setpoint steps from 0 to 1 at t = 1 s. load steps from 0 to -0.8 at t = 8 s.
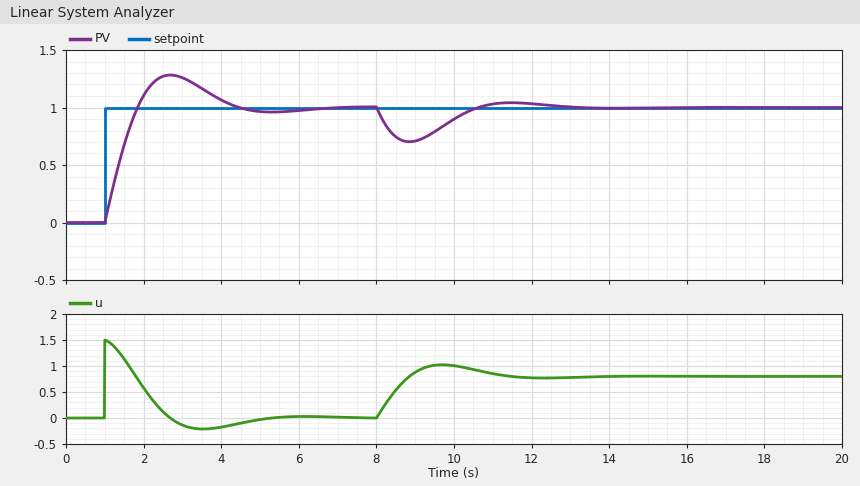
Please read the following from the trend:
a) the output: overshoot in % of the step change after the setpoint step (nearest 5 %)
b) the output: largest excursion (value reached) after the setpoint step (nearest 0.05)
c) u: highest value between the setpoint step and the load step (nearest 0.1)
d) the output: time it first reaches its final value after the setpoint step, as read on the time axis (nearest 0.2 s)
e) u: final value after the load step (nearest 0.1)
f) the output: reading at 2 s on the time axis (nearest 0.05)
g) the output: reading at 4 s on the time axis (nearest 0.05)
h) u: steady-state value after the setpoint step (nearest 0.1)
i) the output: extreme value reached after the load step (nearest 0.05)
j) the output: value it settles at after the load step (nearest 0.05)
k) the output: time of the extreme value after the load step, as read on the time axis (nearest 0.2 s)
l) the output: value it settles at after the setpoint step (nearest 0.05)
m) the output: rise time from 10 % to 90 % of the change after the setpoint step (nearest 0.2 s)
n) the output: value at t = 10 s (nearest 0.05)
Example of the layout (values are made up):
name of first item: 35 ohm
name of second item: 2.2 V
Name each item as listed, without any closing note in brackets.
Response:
the output: overshoot in % of the step change after the setpoint step: 30 %
the output: largest excursion (value reached) after the setpoint step: 1.30
u: highest value between the setpoint step and the load step: 1.5
the output: time it first reaches its final value after the setpoint step, as read on the time axis: 1.8 s
u: final value after the load step: 0.8
the output: reading at 2 s on the time axis: 1.10
the output: reading at 4 s on the time axis: 1.05
u: steady-state value after the setpoint step: 0.0
the output: extreme value reached after the load step: 0.70
the output: value it settles at after the load step: 1.00
the output: time of the extreme value after the load step, as read on the time axis: 8.8 s
the output: value it settles at after the setpoint step: 1.00
the output: rise time from 10 % to 90 % of the change after the setpoint step: 0.6 s
the output: value at t = 10 s: 0.90
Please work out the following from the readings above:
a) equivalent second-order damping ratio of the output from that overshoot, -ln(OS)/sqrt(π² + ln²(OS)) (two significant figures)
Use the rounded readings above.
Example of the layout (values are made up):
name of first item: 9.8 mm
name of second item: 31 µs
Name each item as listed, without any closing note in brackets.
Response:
equivalent second-order damping ratio of the output from that overshoot, -ln(OS)/sqrt(π² + ln²(OS)): 0.36
